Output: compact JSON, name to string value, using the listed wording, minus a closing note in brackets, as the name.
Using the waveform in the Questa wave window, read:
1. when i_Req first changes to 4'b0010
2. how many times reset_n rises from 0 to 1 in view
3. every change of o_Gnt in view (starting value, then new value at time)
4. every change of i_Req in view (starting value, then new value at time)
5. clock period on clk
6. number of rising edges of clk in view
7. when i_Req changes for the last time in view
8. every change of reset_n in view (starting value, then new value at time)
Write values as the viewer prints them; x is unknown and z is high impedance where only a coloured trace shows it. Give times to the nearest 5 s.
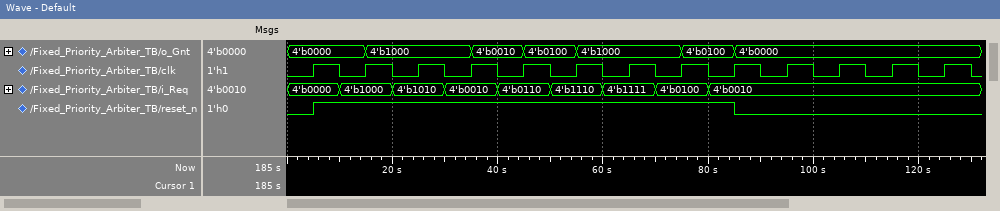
{"when i_Req first changes to 4'b0010": "30 s", "how many times reset_n rises from 0 to 1 in view": "1", "every change of o_Gnt in view": "4'b0000, 4'b1000 at 15 s, 4'b0010 at 35 s, 4'b0100 at 45 s, 4'b1000 at 55 s, 4'b0100 at 75 s, 4'b0000 at 85 s", "every change of i_Req in view": "4'b0000, 4'b1000 at 10 s, 4'b1010 at 20 s, 4'b0010 at 30 s, 4'b0110 at 40 s, 4'b1110 at 50 s, 4'b1111 at 60 s, 4'b0100 at 70 s, 4'b0010 at 80 s", "clock period on clk": "10 s", "number of rising edges of clk in view": "13", "when i_Req changes for the last time in view": "80 s", "every change of reset_n in view": "0, 1 at 5 s, 0 at 85 s"}
